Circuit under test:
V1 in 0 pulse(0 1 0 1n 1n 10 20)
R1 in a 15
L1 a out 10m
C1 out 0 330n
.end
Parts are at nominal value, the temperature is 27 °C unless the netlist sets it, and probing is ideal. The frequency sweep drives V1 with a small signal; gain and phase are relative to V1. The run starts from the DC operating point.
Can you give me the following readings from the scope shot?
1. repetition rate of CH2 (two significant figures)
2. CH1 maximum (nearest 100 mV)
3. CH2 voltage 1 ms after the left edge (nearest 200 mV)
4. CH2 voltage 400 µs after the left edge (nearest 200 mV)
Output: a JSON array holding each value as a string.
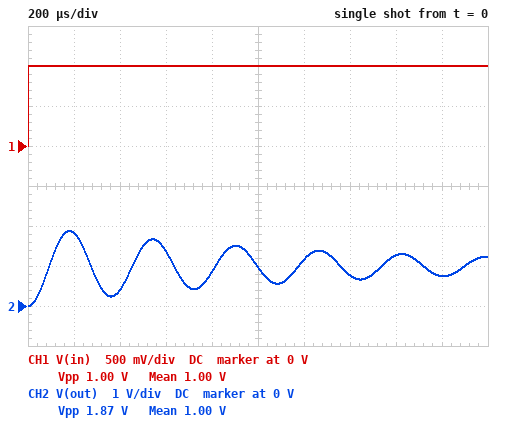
["2.8 kHz", "1.0 V", "1.0 V", "400 mV"]
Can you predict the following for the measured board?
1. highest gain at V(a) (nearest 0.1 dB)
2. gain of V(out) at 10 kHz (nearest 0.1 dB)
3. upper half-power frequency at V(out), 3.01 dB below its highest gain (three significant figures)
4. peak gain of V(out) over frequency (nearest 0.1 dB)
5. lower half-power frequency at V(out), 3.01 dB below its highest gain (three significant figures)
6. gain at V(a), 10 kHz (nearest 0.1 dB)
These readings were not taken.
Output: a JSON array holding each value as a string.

["0 dB", "-21.6 dB", "2.88 kHz", "21.3 dB", "2.64 kHz", "0 dB"]
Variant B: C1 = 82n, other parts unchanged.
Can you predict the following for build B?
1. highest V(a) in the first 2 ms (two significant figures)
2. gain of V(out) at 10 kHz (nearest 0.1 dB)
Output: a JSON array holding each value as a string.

["1.0 V", "-7.0 dB"]
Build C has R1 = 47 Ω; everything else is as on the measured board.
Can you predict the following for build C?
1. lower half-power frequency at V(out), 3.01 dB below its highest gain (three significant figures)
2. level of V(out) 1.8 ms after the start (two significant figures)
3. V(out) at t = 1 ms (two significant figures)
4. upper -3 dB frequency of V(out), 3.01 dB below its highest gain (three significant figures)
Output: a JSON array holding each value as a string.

["2.31 kHz", "990 mV", "1.0 V", "3.07 kHz"]
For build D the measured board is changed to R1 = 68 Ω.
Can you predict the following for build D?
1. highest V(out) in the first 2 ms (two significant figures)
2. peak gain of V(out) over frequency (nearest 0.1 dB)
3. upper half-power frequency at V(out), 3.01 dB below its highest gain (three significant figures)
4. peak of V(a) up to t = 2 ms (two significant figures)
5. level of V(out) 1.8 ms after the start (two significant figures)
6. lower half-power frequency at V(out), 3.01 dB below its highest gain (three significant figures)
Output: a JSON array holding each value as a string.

["1.5 V", "8.3 dB", "3.17 kHz", "1.2 V", "1.0 V", "2.04 kHz"]
